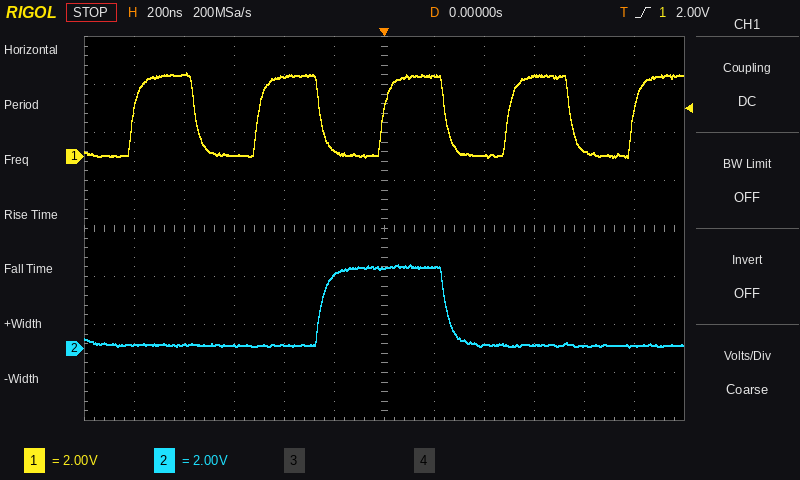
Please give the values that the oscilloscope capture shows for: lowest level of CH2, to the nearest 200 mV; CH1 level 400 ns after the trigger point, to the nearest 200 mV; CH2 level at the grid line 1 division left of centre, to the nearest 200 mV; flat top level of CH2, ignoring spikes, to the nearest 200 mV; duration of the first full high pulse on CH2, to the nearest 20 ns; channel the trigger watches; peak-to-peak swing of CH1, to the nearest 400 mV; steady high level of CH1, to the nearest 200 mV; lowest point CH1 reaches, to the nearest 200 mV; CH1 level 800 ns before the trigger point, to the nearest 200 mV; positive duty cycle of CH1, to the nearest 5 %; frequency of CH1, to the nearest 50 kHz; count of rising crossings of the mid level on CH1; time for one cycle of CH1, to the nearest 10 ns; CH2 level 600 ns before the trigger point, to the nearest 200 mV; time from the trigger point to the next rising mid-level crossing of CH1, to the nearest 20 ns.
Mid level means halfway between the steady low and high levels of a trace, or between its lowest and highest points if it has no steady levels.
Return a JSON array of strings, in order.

["0.0 V", "0.0 V", "3.0 V", "3.4 V", "500 ns", "CH1", "3.6 V", "3.4 V", "0.0 V", "3.4 V", "50 %", "2.00 MHz", "5", "500 ns", "200 mV", "500 ns"]
